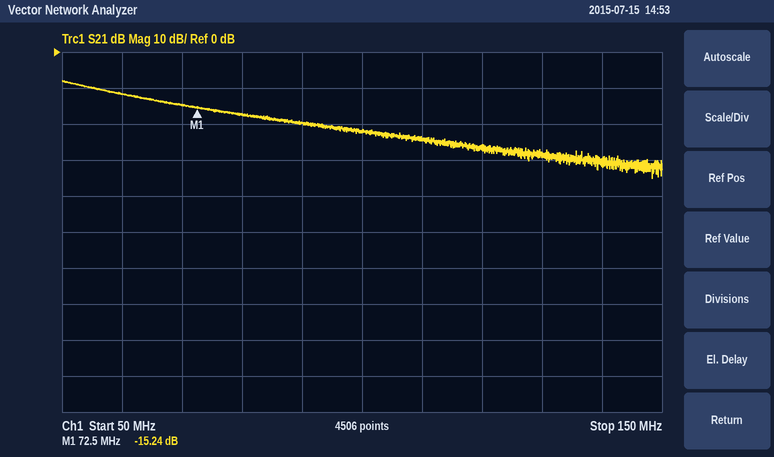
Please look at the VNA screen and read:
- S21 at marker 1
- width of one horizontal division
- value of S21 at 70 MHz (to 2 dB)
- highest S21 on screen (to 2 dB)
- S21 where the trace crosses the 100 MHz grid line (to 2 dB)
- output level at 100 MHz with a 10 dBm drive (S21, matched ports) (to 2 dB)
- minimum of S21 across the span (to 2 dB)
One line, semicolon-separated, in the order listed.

-15.24 dB; 10 MHz; -14 dB; -8 dB; -22 dB; -12 dBm; -36 dB
